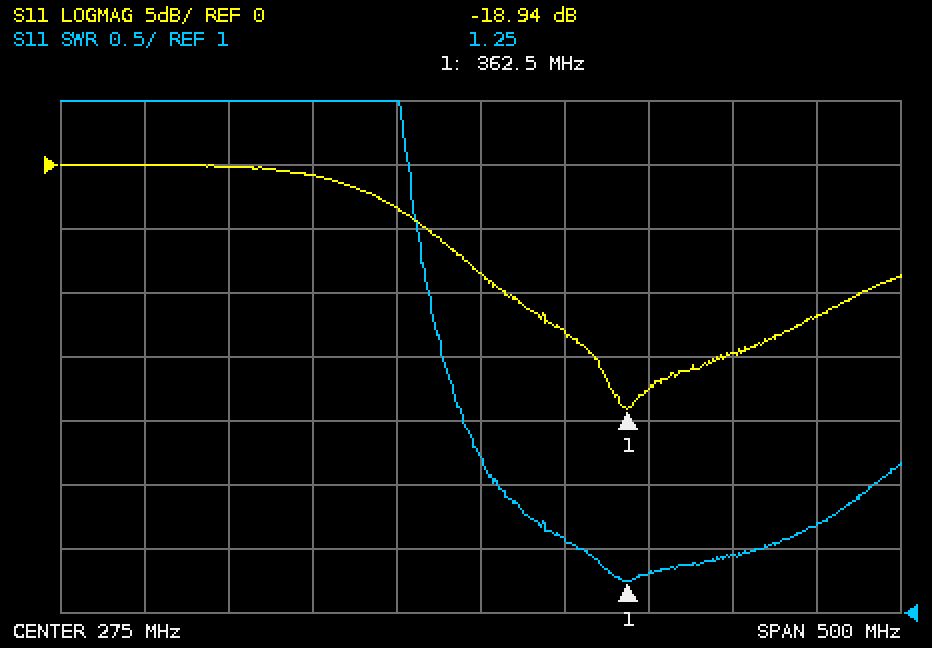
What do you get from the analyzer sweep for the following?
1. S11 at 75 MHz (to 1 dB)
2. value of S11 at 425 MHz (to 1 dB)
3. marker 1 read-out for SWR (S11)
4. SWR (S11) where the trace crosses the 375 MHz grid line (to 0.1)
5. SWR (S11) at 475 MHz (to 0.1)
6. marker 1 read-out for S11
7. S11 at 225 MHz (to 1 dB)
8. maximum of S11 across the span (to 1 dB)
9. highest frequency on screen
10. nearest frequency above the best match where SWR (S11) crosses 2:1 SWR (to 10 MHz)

0 dB
-15 dB
1.25
1.3
1.7
-18.94 dB
-3 dB
0 dB
525 MHz
510 MHz
